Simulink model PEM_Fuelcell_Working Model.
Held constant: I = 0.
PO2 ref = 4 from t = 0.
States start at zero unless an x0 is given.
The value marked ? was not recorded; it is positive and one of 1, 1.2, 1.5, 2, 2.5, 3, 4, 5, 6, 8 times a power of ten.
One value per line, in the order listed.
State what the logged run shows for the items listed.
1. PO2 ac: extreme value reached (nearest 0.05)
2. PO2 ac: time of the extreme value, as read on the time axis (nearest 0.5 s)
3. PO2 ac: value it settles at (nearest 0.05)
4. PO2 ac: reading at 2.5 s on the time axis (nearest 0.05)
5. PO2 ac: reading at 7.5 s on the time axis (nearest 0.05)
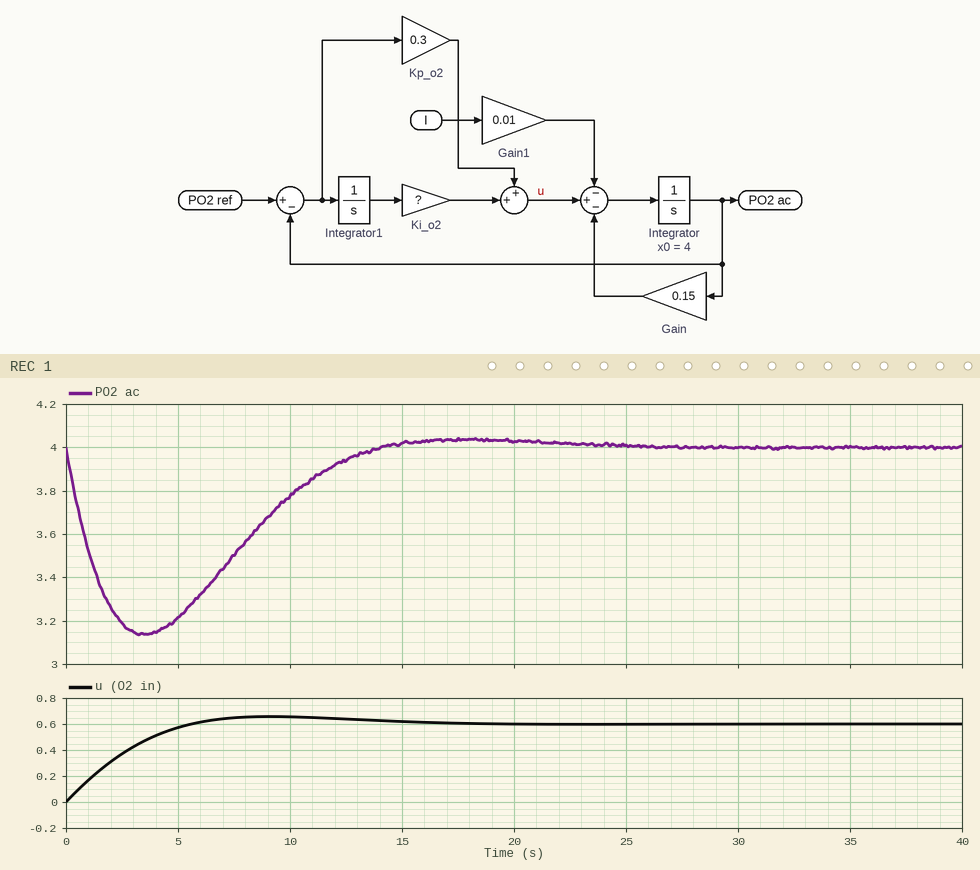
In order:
3.15
3.5 s
4.00
3.20
3.50
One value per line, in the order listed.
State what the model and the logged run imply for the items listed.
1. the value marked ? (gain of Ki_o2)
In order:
0.1
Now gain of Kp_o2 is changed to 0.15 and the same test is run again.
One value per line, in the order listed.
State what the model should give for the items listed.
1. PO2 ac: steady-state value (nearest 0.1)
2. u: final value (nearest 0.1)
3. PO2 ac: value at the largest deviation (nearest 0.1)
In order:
4.0
0.6
2.9
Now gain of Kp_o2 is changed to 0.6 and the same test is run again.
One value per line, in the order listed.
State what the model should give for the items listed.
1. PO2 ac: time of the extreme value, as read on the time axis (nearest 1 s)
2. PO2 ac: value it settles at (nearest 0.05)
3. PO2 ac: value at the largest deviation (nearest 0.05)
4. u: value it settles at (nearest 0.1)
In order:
3 s
4.00
3.40
0.6
